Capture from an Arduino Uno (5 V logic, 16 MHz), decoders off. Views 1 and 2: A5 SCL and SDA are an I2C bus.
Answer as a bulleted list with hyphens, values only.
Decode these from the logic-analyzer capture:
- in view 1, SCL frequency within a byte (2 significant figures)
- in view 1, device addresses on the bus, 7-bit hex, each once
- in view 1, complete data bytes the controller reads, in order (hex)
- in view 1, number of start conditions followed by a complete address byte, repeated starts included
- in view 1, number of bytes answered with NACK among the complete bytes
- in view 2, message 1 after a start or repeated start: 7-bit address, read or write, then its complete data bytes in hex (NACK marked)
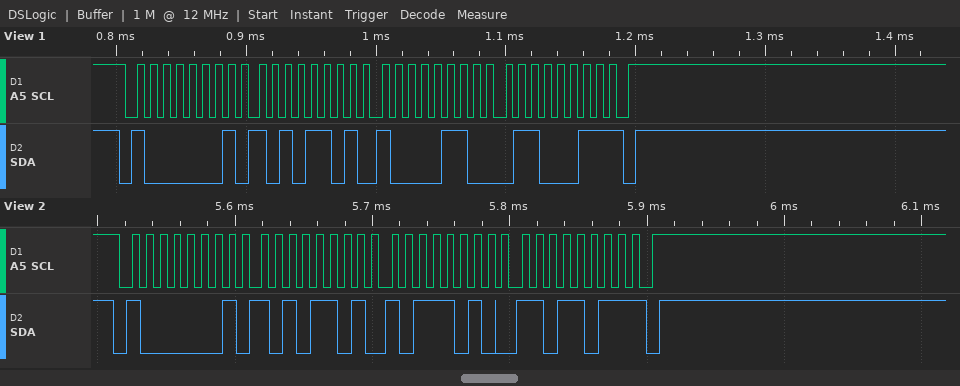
- 100 kHz
- 0x40
- AD 86 63
- 1
- 1
- 0x40 read: AD BA DB NACK
